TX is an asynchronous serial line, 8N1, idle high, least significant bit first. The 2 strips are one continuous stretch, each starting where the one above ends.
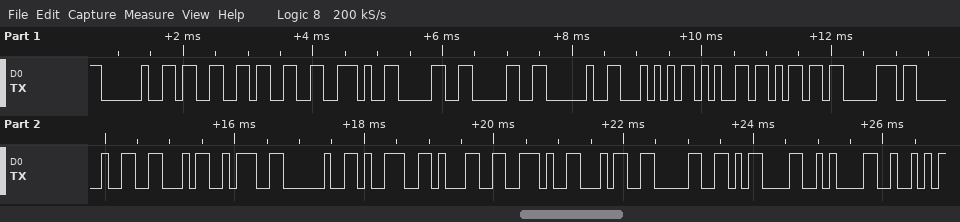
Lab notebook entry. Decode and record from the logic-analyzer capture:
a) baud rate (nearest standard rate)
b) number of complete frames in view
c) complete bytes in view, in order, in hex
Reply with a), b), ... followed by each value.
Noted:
a) 9600 baud
b) 23
c) 20 33 33 2E 30 30 20 54 65 6D 70 20 46 3A 20 39 31 2E 34 30 0D 0A 52
